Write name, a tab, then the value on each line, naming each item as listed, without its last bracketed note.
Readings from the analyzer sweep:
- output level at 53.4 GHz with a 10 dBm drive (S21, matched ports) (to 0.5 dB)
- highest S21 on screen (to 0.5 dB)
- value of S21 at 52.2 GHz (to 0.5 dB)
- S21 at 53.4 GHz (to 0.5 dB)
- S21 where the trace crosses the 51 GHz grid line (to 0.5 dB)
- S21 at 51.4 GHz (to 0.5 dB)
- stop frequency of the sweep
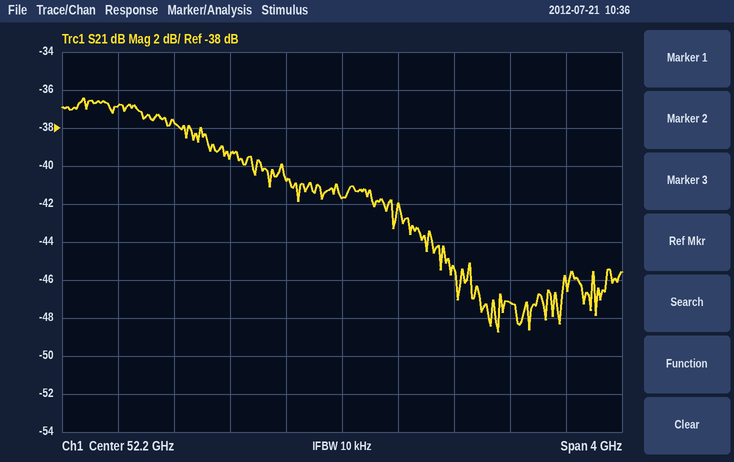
output level at 53.4 GHz with a 10 dBm drive (S21, matched ports)	-37.0 dBm
highest S21 on screen	-36.5 dB
value of S21 at 52.2 GHz	-41.5 dB
S21 at 53.4 GHz	-47.0 dB
S21 where the trace crosses the 51 GHz grid line	-37.5 dB
S21 at 51.4 GHz	-39.5 dB
stop frequency of the sweep	54.2 GHz
